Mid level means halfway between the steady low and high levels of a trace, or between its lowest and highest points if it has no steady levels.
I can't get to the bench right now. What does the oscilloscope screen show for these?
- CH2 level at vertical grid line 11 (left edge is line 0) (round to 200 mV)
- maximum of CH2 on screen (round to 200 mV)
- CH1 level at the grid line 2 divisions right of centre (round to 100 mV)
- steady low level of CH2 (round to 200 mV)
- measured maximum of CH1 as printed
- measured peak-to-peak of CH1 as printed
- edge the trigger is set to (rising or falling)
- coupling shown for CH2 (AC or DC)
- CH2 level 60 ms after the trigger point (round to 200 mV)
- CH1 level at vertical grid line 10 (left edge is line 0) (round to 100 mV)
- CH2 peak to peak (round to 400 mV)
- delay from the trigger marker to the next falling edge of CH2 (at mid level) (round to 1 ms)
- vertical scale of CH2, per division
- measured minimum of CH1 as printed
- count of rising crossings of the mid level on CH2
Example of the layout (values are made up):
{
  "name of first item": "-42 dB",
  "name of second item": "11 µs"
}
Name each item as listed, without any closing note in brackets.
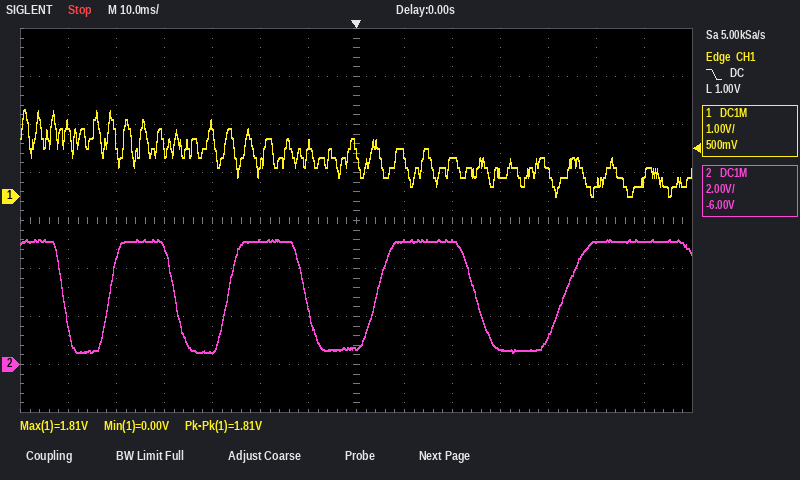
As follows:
{
  "CH2 level at vertical grid line 11 (left edge is line 0)": "1.2 V",
  "maximum of CH2 on screen": "5.2 V",
  "CH1 level at the grid line 2 divisions right of centre": "800 mV",
  "steady low level of CH2": "600 mV",
  "measured maximum of CH1 as printed": "1.81 V",
  "measured peak-to-peak of CH1 as printed": "1.81 V",
  "edge the trigger is set to": "falling",
  "coupling shown for CH2": "DC",
  "CH2 level 60 ms after the trigger point": "5.2 V",
  "CH1 level at vertical grid line 10 (left edge is line 0)": "500 mV",
  "CH2 peak to peak": "4.8 V",
  "delay from the trigger marker to the next falling edge of CH2 (at mid level)": "25 ms",
  "vertical scale of CH2, per division": "2 V",
  "measured minimum of CH1 as printed": "0.00 V",
  "count of rising crossings of the mid level on CH2": "4"
}
